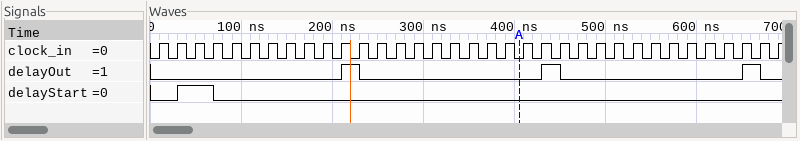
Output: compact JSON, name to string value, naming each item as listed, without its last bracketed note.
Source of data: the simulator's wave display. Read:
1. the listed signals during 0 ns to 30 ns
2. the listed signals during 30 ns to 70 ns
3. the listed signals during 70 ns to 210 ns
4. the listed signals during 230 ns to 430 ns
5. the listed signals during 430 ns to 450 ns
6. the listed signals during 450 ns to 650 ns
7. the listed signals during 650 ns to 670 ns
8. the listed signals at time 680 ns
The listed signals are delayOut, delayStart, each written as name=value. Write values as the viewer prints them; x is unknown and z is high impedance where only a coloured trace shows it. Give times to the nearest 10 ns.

{"the listed signals during 0 ns to 30 ns": "delayOut=0, delayStart=0", "the listed signals during 30 ns to 70 ns": "delayOut=0, delayStart=1", "the listed signals during 70 ns to 210 ns": "delayOut=0, delayStart=0", "the listed signals during 230 ns to 430 ns": "delayOut=0, delayStart=0", "the listed signals during 430 ns to 450 ns": "delayOut=1, delayStart=0", "the listed signals during 450 ns to 650 ns": "delayOut=0, delayStart=0", "the listed signals during 650 ns to 670 ns": "delayOut=1, delayStart=0", "the listed signals at time 680 ns": "delayOut=0, delayStart=0"}
